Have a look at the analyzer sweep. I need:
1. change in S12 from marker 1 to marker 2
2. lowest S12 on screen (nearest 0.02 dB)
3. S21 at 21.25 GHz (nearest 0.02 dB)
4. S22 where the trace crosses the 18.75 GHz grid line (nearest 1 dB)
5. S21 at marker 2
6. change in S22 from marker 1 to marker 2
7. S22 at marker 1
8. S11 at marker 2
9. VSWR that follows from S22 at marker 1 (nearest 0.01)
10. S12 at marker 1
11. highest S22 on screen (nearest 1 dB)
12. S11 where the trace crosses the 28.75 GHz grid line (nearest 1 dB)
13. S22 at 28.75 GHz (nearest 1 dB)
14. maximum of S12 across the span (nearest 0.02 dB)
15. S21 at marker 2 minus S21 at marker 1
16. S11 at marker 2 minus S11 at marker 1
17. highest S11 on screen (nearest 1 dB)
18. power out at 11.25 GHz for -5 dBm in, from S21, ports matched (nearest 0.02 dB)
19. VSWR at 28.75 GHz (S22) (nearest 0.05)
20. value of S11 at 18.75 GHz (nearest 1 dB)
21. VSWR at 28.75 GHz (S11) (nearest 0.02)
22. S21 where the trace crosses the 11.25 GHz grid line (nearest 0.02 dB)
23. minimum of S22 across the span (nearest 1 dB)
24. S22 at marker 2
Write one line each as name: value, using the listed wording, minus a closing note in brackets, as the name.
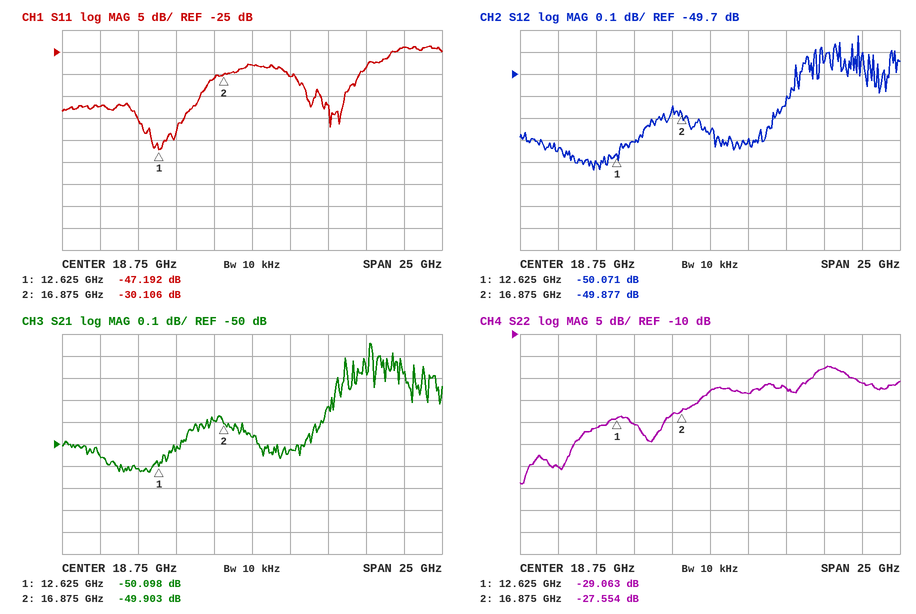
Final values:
change in S12 from marker 1 to marker 2: 0.194 dB
lowest S12 on screen: -50.14 dB
S21 at 21.25 GHz: -50.02 dB
S22 where the trace crosses the 18.75 GHz grid line: -23 dB
S21 at marker 2: -49.903 dB
change in S22 from marker 1 to marker 2: 1.509 dB
S22 at marker 1: -29.063 dB
S11 at marker 2: -30.106 dB
VSWR that follows from S22 at marker 1: 1.07
S12 at marker 1: -50.071 dB
highest S22 on screen: -17 dB
S11 where the trace crosses the 28.75 GHz grid line: -24 dB
S22 at 28.75 GHz: -21 dB
maximum of S12 across the span: -49.52 dB
S21 at marker 2 minus S21 at marker 1: 0.195 dB
S11 at marker 2 minus S11 at marker 1: 17.086 dB
highest S11 on screen: -24 dB
power out at 11.25 GHz for -5 dBm in, from S21, ports matched: -55.12 dBm
VSWR at 28.75 GHz (S22): 1.20
value of S11 at 18.75 GHz: -28 dB
VSWR at 28.75 GHz (S11): 1.14
S21 where the trace crosses the 11.25 GHz grid line: -50.12 dB
minimum of S22 across the span: -44 dB
S22 at marker 2: -27.554 dB
